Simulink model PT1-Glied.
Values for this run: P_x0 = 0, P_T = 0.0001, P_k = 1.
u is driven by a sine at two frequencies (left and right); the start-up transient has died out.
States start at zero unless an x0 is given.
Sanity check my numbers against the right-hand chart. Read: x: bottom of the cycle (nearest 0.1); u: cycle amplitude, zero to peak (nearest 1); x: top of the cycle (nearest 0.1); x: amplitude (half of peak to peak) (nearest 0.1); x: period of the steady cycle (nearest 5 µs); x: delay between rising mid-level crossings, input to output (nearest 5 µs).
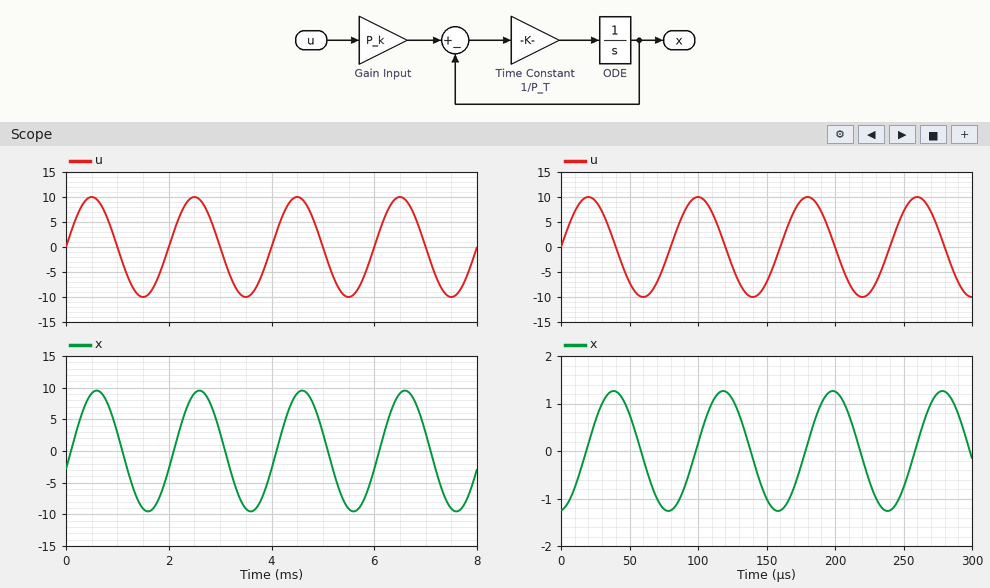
-1.3
10
1.3
1.3
80 µs
20 µs
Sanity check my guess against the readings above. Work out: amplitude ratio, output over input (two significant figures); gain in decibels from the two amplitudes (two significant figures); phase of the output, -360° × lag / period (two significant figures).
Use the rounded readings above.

0.13
-18 dB
-90°
